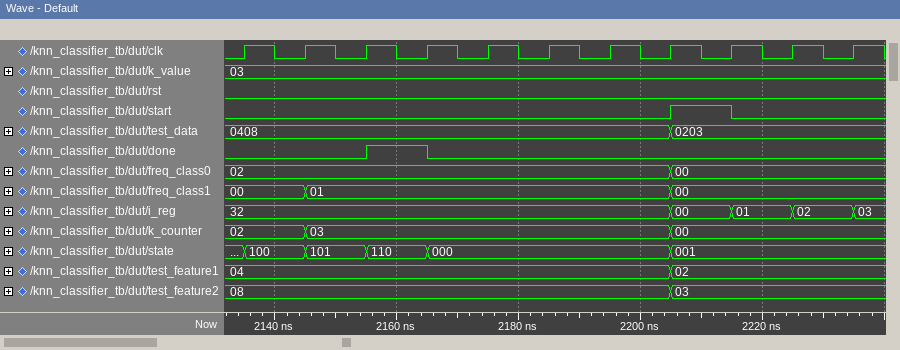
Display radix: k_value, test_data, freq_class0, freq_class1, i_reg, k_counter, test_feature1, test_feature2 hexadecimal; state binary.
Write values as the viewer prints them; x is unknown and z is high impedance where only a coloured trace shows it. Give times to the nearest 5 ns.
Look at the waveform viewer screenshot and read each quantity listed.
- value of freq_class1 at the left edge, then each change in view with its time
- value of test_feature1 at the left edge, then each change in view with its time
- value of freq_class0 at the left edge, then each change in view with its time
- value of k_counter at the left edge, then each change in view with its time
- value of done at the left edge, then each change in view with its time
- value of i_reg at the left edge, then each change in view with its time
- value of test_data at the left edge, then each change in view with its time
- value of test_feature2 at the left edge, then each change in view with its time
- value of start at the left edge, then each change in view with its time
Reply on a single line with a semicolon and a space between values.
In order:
00, 01 at 2145 ns, 00 at 2205 ns; 04, 02 at 2205 ns; 02, 00 at 2205 ns; 02, 03 at 2145 ns, 00 at 2205 ns; 0, 1 at 2155 ns, 0 at 2165 ns; 32, 00 at 2205 ns, 01 at 2215 ns, 02 at 2225 ns, 03 at 2235 ns; 0408, 0203 at 2205 ns; 08, 03 at 2205 ns; 0, 1 at 2205 ns, 0 at 2215 ns
